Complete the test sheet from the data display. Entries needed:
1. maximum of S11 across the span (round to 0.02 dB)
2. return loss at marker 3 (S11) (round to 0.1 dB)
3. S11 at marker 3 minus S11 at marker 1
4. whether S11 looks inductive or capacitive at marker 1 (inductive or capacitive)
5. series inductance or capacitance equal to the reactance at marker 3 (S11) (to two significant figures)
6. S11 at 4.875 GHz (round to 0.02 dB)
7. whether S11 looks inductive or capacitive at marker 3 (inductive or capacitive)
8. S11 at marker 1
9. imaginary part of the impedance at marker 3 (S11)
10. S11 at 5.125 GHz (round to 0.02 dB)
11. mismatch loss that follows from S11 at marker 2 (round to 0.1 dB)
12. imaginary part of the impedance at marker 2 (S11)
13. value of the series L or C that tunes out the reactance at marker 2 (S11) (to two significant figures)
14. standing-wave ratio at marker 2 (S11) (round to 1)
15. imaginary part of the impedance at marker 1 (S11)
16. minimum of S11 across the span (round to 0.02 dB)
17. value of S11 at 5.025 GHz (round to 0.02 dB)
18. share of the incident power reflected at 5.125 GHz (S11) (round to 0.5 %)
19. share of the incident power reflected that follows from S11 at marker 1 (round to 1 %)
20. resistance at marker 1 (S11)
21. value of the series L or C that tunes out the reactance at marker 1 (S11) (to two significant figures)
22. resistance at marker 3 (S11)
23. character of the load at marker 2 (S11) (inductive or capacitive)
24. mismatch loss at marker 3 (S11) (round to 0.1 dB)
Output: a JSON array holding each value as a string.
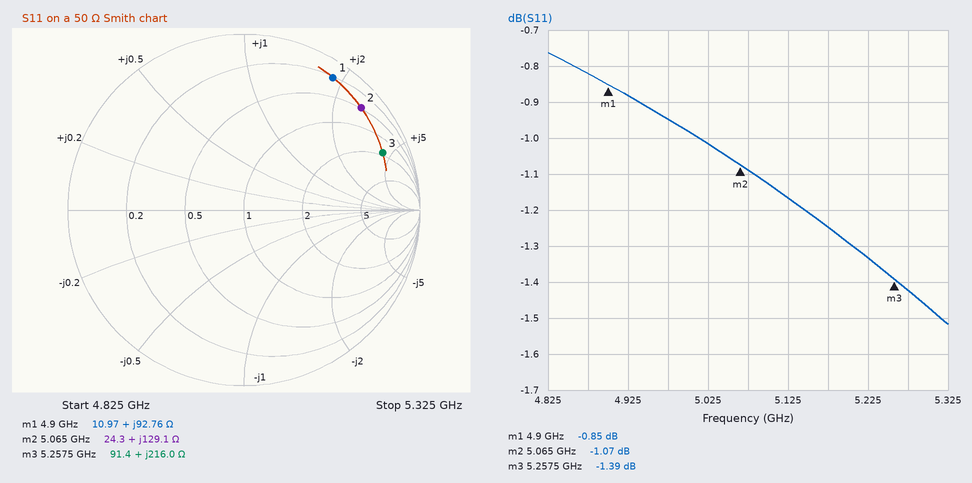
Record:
["-0.76 dB", "1.4 dB", "-0.54 dB", "inductive", "6.5 nH", "-0.82 dB", "inductive", "-0.85 dB", "+216.0 Ω", "-1.16 dB", "6.6 dB", "+129.1 Ω", "240 fF", "16", "+92.76 Ω", "-1.52 dB", "-1.02 dB", "76.5 %", "82 %", "10.97 Ω", "350 fF", "91.4 Ω", "inductive", "5.6 dB"]
